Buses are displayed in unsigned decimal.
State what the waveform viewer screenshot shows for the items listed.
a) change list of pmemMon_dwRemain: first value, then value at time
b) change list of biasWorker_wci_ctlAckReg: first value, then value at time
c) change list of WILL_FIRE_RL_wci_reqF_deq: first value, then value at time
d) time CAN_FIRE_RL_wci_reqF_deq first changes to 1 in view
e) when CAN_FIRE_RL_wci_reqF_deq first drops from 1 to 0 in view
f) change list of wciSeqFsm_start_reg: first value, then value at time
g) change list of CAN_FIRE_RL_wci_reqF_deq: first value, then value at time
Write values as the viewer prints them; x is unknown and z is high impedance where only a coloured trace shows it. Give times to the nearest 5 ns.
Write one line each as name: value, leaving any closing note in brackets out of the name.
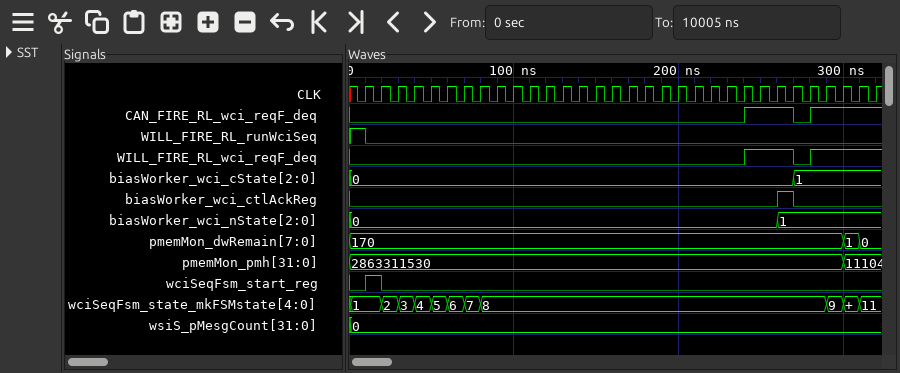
change list of pmemMon_dwRemain: first value, then value at time: 170, 1 at 300 ns, 0 at 310 ns
change list of biasWorker_wci_ctlAckReg: first value, then value at time: 0, 1 at 260 ns, 0 at 270 ns
change list of WILL_FIRE_RL_wci_reqF_deq: first value, then value at time: 0, 1 at 240 ns, 0 at 270 ns, 1 at 280 ns
time CAN_FIRE_RL_wci_reqF_deq first changes to 1 in view: 240 ns
when CAN_FIRE_RL_wci_reqF_deq first drops from 1 to 0 in view: 270 ns
change list of wciSeqFsm_start_reg: first value, then value at time: 0, 1 at 10 ns, 0 at 20 ns
change list of CAN_FIRE_RL_wci_reqF_deq: first value, then value at time: 0, 1 at 240 ns, 0 at 270 ns, 1 at 280 ns
